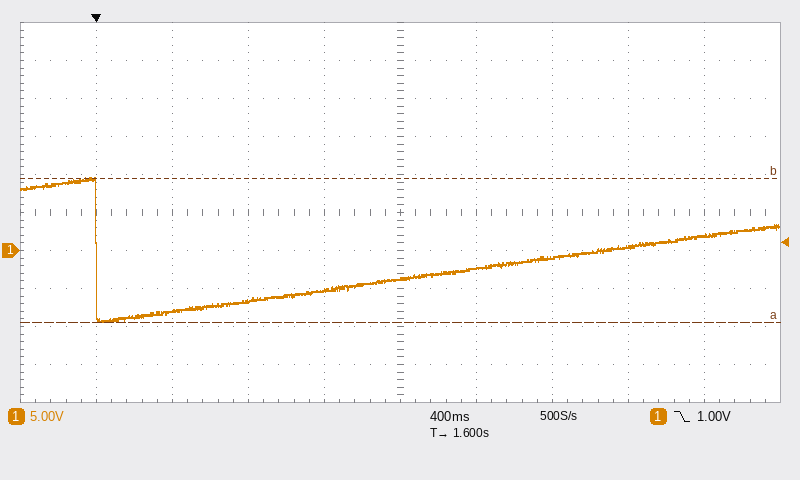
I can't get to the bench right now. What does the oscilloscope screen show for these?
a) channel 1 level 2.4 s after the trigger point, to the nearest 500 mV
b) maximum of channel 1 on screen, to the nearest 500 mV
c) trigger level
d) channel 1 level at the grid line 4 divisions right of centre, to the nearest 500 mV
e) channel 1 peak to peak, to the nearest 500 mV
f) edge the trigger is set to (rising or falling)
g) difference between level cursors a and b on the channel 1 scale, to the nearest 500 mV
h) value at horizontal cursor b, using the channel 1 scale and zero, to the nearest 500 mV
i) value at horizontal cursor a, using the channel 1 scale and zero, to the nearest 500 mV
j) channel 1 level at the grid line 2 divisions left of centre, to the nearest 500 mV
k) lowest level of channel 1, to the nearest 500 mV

-1.0 V
9.5 V
1.00 V
2.0 V
19.0 V
falling
19.0 V
9.5 V
-9.5 V
-6.5 V
-9.5 V
